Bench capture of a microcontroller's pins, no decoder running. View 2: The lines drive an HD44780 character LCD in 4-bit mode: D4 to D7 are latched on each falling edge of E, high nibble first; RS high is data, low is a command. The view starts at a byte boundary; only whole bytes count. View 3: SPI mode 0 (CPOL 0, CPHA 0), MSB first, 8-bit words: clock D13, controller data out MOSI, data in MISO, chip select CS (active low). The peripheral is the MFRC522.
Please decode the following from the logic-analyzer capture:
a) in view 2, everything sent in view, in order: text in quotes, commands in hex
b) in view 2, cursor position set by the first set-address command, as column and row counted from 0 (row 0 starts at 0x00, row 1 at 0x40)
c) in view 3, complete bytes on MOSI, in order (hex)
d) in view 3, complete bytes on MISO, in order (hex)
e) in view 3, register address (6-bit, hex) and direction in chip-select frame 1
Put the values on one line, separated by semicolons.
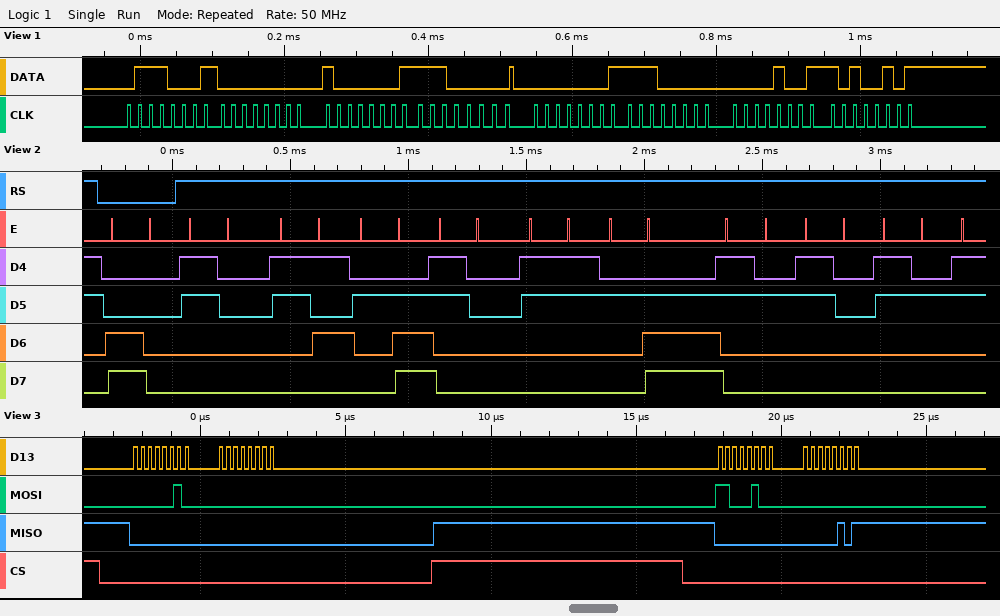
0xC0 "05.03.202"; column 0, row 1; 02 00 C4 00; 00 00 00 05; 0x01 write
